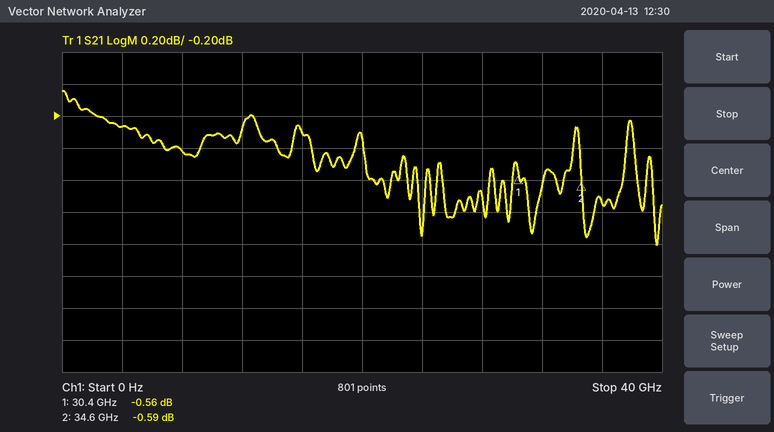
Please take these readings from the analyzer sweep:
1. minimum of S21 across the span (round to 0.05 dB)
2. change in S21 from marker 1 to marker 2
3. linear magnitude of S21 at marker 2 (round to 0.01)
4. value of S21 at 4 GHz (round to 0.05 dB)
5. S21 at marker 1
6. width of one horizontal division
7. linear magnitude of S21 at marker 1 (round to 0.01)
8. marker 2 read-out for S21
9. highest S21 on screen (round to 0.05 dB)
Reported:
-1.00 dB
-0.03 dB
0.93
-0.25 dB
-0.56 dB
4 GHz
0.94
-0.59 dB
-0.05 dB
